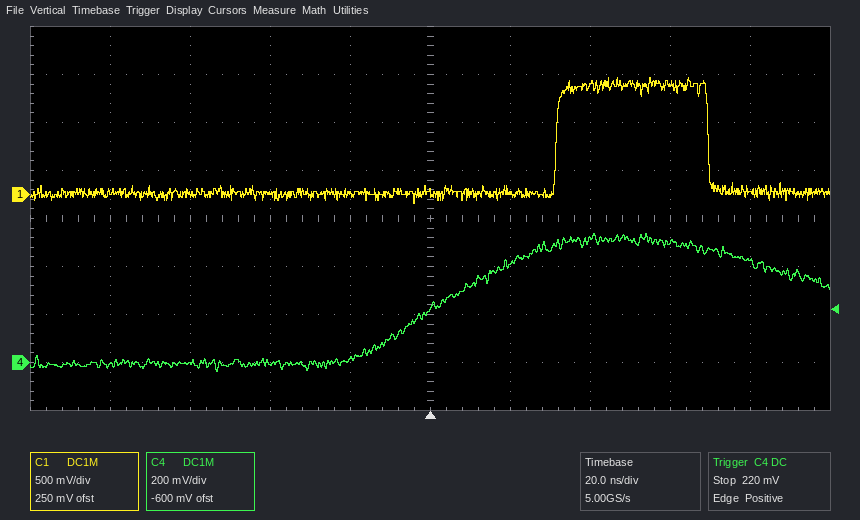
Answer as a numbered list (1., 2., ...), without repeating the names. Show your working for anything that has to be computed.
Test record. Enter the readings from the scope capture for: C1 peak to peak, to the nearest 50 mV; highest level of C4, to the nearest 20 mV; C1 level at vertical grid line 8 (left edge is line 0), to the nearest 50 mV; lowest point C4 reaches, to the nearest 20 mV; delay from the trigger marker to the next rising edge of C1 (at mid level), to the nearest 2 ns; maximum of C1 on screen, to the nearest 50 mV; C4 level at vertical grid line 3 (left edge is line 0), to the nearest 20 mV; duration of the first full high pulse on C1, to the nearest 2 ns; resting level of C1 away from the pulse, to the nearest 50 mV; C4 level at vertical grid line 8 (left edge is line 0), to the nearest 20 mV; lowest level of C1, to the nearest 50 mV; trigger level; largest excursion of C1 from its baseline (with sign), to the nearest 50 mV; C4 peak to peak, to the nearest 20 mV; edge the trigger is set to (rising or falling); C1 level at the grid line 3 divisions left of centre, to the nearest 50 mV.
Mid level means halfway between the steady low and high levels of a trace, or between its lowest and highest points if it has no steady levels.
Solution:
1. 1.20 V − (-100 mV) = 1.30 V
2. 540 mV
3. 1.15 V
4. -40 mV
5. 32 ns
6. 1.20 V
7. 0 mV
8. 38 ns
9. 0 mV
10. 500 mV
11. -100 mV
12. 220 mV
13. 1.20 V − (0 mV) = +1.20 V
14. 540 mV − (-40 mV) = 580 mV
15. rising
16. 0 mV
